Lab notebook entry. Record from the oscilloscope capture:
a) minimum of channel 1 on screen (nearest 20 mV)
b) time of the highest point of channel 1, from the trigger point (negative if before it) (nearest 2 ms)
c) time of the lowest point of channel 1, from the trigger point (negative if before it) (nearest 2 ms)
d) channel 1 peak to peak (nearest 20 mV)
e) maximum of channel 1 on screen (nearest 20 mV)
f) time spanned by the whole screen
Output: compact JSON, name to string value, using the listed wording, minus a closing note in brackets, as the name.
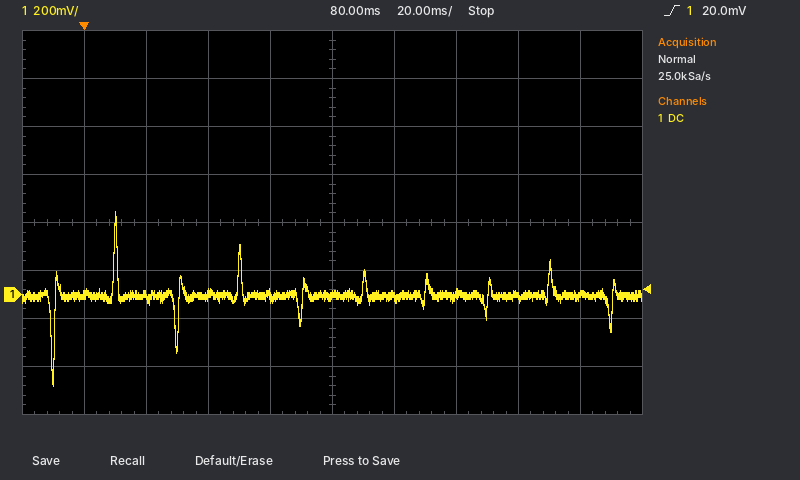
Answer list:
{"minimum of channel 1 on screen": "-380 mV", "time of the highest point of channel 1, from the trigger point (negative if before it)": "+10 ms", "time of the lowest point of channel 1, from the trigger point (negative if before it)": "-10 ms", "channel 1 peak to peak": "720 mV", "maximum of channel 1 on screen": "340 mV", "time spanned by the whole screen": "200 ms"}
